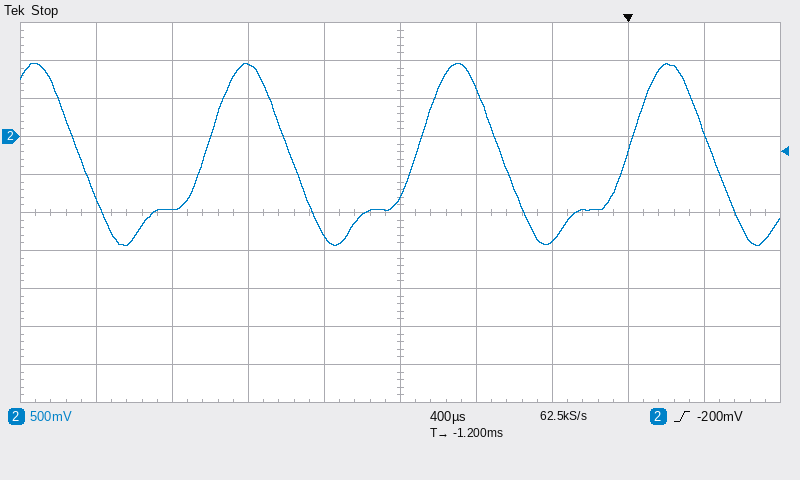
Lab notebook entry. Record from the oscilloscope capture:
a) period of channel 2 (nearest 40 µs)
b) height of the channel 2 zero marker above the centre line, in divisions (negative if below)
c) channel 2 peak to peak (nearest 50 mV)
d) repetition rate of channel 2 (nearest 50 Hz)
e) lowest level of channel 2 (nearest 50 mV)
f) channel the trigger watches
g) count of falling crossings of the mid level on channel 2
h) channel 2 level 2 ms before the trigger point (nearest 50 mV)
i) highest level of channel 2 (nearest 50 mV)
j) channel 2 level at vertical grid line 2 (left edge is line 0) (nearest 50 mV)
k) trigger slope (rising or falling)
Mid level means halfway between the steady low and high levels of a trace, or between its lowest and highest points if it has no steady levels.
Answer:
1.12 ms
+2.0 div
2.40 V
900 Hz
-1.45 V
channel 2
4
950 mV
950 mV
-950 mV
rising
